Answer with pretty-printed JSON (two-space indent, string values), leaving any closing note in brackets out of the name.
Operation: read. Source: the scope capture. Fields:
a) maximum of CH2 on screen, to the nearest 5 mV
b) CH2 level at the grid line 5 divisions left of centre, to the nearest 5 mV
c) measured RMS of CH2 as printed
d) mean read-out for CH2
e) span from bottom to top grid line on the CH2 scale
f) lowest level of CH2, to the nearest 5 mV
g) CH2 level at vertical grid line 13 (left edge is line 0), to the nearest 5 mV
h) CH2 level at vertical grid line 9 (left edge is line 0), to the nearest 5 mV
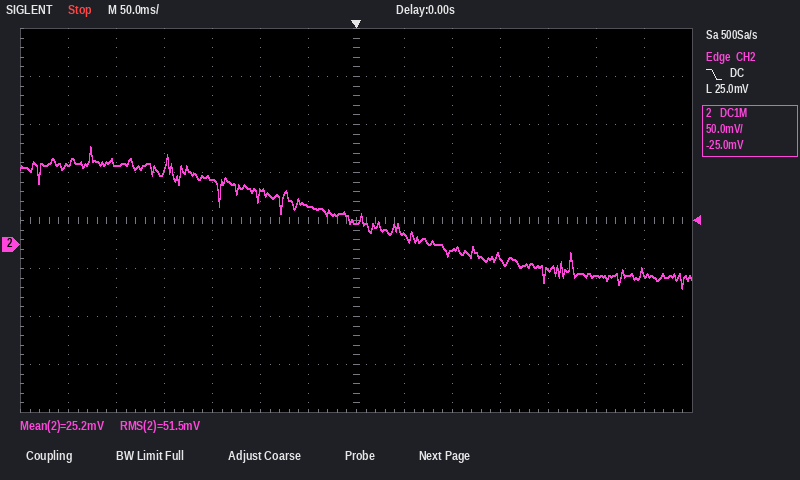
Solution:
{
  "maximum of CH2 on screen, to the nearest 5 mV": "100 mV",
  "CH2 level at the grid line 5 divisions left of centre, to the nearest 5 mV": "80 mV",
  "measured RMS of CH2 as printed": "51.5 mV",
  "mean read-out for CH2": "25.2 mV",
  "span from bottom to top grid line on the CH2 scale": "400 mV",
  "lowest level of CH2, to the nearest 5 mV": "-45 mV",
  "CH2 level at vertical grid line 13 (left edge is line 0), to the nearest 5 mV": "-30 mV",
  "CH2 level at vertical grid line 9 (left edge is line 0), to the nearest 5 mV": "-5 mV"
}
